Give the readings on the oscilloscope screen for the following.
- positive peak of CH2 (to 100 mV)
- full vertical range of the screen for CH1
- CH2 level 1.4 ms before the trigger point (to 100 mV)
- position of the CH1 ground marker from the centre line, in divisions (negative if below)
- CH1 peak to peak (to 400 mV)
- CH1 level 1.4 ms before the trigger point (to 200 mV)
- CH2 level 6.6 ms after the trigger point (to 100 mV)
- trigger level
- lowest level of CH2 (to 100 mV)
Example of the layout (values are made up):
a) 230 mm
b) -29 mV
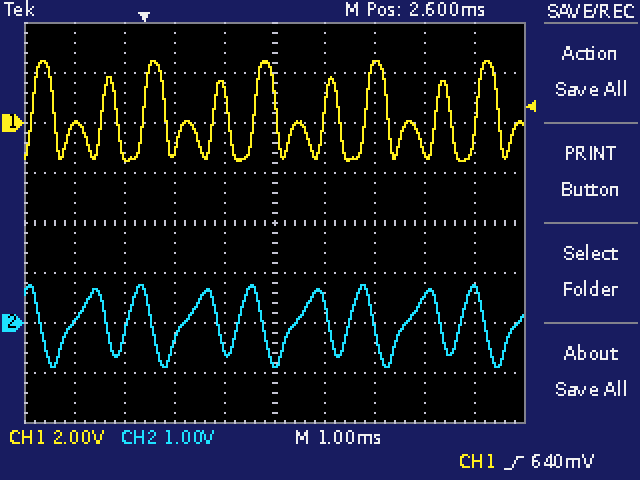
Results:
a) 800 mV
b) 16 V
c) 0.0 V
d) +2.0 div
e) 4.0 V
f) 0.0 V
g) 700 mV
h) 640 mV
i) -900 mV
